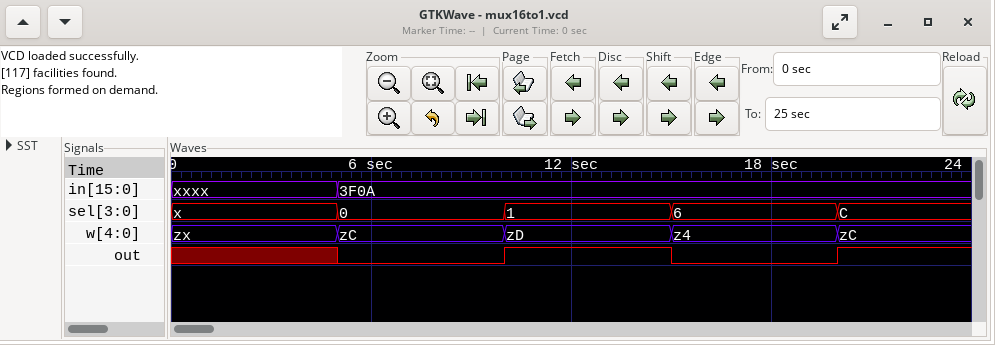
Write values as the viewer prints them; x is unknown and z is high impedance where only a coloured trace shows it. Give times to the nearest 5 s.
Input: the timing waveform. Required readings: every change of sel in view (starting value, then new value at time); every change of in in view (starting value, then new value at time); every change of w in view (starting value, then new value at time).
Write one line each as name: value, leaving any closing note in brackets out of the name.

every change of sel in view: x, 0 at 5 s, 1 at 10 s, 6 at 15 s, C at 20 s
every change of in in view: xxxx, 3F0A at 5 s
every change of w in view: zx, zC at 5 s, zD at 10 s, z4 at 15 s, zC at 20 s
